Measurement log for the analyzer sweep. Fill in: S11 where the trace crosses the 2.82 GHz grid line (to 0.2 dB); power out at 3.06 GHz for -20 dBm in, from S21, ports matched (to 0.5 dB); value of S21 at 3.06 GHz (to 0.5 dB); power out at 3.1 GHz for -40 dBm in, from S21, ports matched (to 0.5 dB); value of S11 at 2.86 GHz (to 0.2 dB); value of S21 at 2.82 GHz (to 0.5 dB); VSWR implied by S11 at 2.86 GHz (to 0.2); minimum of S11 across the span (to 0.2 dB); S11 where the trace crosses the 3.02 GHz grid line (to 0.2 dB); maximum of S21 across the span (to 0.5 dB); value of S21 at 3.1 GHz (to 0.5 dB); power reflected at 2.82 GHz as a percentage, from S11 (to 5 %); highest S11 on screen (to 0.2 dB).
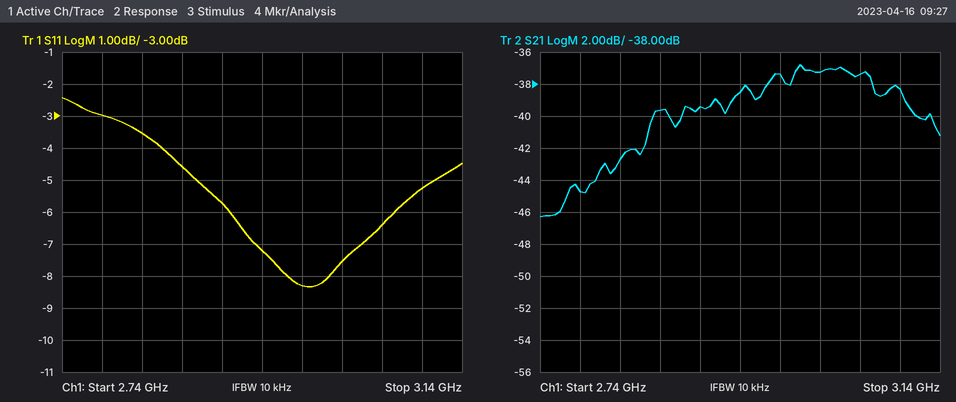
-3.6 dB
-57.5 dBm
-37.5 dB
-78.5 dBm
-4.6 dB
-42.5 dB
3.8
-8.4 dB
-7.6 dB
-37.0 dB
-38.5 dB
45 %
-2.4 dB
